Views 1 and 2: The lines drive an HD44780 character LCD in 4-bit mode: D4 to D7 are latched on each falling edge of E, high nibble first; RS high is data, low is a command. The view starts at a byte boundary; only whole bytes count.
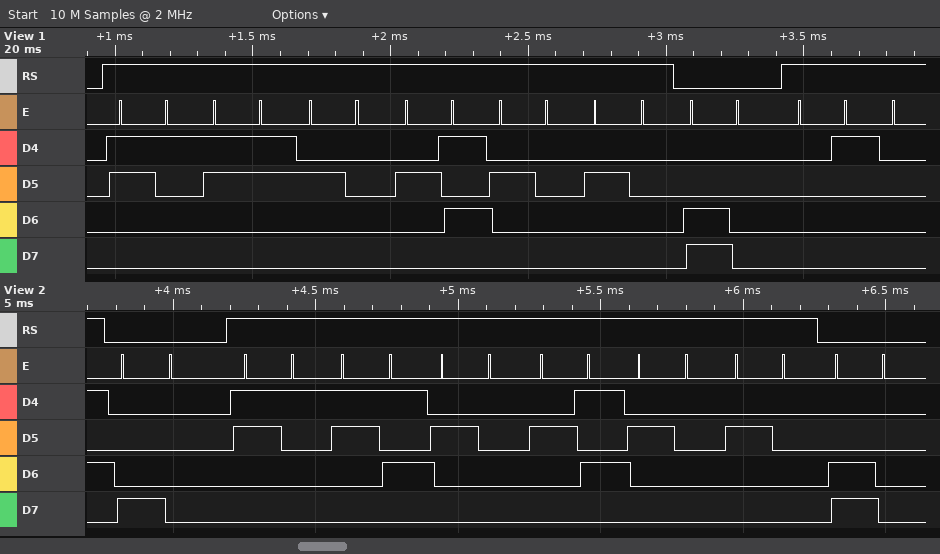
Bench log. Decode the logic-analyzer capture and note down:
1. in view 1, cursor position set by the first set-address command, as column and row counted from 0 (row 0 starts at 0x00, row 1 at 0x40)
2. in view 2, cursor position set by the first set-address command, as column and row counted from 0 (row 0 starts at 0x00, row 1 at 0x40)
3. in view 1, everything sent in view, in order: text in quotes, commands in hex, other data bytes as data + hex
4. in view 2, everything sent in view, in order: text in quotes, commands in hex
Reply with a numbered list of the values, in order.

1. column 0, row 1
2. column 0, row 0
3. "13 %  " 0xC0 data 01
4. 0x80 "15 %  " 0xC0
